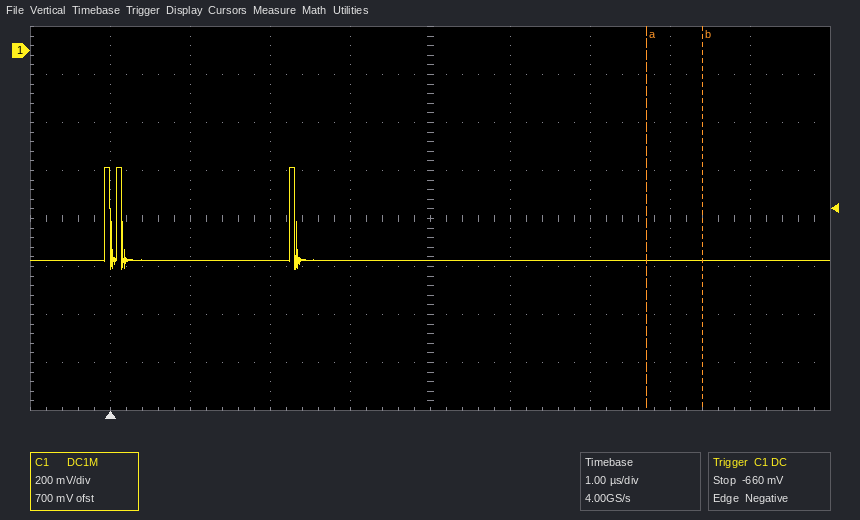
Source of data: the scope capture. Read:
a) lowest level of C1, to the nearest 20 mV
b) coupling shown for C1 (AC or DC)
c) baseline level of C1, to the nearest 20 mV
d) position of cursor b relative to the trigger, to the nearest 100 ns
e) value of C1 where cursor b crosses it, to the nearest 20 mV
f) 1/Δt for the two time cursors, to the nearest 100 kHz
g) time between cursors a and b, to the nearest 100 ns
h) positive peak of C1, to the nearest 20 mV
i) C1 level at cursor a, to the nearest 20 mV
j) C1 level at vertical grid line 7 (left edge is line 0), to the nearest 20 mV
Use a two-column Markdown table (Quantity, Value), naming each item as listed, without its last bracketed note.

| Quantity | Value |
|---|---|
| lowest level of C1, to the nearest 20 mV | -920 mV |
| coupling shown for C1 | DC |
| baseline level of C1, to the nearest 20 mV | -880 mV |
| position of cursor b relative to the trigger, to the nearest 100 ns | +7.4 µs |
| value of C1 where cursor b crosses it, to the nearest 20 mV | -880 mV |
| 1/Δt for the two time cursors, to the nearest 100 kHz | 1.4 MHz |
| time between cursors a and b, to the nearest 100 ns | 700 ns |
| positive peak of C1, to the nearest 20 mV | -480 mV |
| C1 level at cursor a, to the nearest 20 mV | -880 mV |
| C1 level at vertical grid line 7 (left edge is line 0), to the nearest 20 mV | -880 mV |
